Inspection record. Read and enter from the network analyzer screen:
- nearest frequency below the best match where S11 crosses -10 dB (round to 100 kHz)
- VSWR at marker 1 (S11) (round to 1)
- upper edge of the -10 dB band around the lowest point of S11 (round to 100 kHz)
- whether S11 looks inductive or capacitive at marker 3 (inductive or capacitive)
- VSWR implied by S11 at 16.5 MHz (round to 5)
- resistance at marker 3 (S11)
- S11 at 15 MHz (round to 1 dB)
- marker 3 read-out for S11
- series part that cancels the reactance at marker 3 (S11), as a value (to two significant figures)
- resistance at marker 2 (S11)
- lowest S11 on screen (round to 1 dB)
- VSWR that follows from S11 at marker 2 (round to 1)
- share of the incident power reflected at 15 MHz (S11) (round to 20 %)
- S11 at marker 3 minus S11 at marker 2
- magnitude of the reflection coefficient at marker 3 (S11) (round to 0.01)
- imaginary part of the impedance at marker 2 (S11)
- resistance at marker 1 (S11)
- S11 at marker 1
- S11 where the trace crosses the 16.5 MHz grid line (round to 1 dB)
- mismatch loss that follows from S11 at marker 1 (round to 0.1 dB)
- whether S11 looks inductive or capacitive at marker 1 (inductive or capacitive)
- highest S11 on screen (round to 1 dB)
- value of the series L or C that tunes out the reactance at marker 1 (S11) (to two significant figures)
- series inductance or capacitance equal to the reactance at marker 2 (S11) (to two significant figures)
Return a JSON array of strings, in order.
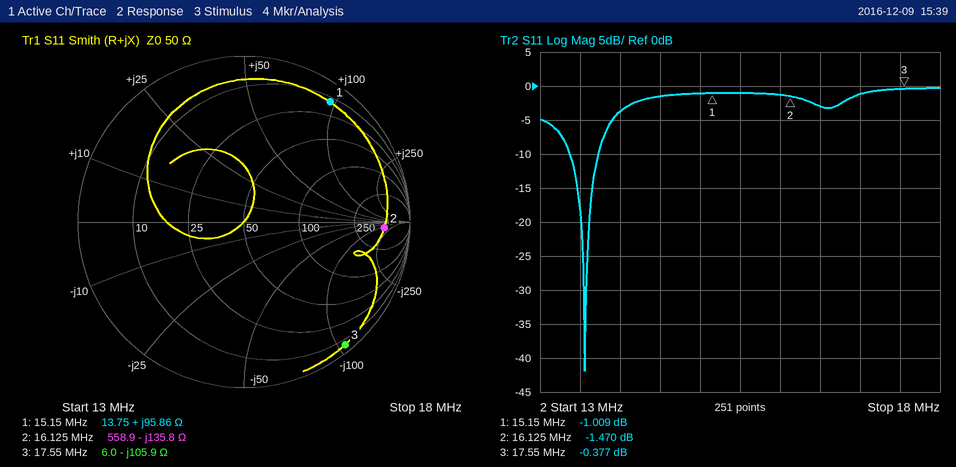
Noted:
["13.4 MHz", "17", "13.7 MHz", "capacitive", "5", "6.0 Ω", "-1 dB", "-0.377 dB", "960 nH", "558.9 Ω", "-42 dB", "12", "80 %", "1.093 dB", "0.96", "-135.8 Ω", "13.75 Ω", "-1.009 dB", "-3 dB", "6.8 dB", "inductive", "0 dB", "110 pF", "73 pF"]
